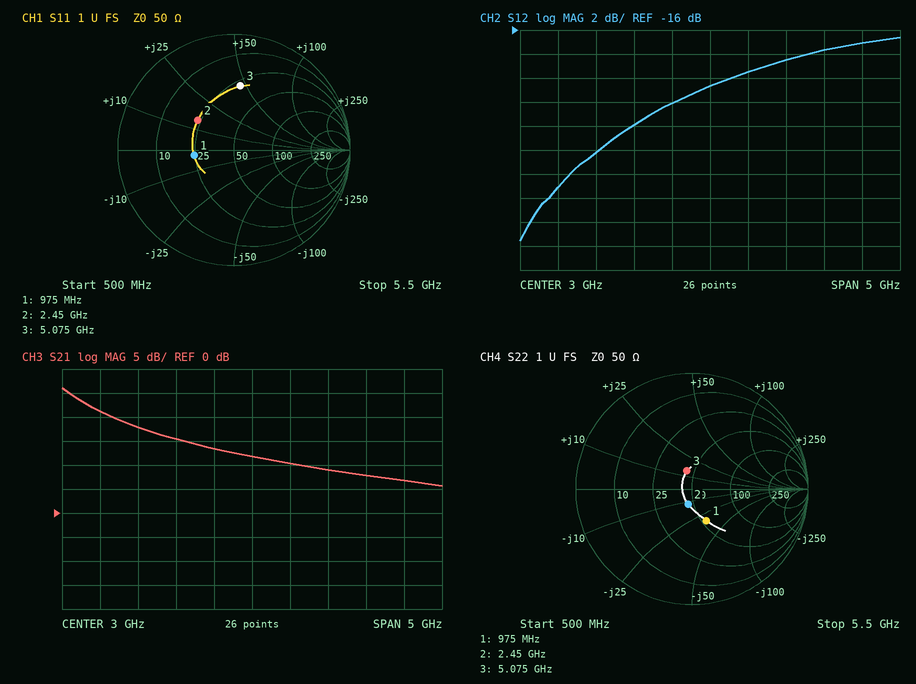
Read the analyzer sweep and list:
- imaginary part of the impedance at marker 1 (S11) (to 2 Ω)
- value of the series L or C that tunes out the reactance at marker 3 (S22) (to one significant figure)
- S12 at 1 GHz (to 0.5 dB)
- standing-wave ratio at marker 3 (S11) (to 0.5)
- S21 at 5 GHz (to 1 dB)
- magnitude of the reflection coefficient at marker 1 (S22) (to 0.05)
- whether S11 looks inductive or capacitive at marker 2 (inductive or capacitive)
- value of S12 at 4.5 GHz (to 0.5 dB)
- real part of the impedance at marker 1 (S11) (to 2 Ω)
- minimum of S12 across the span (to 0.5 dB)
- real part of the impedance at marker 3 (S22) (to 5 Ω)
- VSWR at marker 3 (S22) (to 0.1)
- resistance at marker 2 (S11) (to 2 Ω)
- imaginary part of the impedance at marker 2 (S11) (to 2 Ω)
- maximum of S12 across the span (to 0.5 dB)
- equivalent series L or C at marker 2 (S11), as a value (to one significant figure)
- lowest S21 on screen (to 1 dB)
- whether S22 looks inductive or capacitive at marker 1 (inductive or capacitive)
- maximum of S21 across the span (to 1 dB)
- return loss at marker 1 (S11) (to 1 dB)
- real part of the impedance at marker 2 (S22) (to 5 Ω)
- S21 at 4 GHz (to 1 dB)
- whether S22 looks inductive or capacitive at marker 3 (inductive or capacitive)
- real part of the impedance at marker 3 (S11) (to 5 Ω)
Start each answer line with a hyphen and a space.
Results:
- -2 Ω
- 2 pF
- -29.0 dB
- 3.5
- 7 dB
- 0.30
- inductive
- -17.5 dB
- 24 Ω
- -33.5 dB
- 45 Ω
- 1.4
- 24 Ω
- +14 Ω
- -16.5 dB
- 900 pH
- 6 dB
- capacitive
- 26 dB
- 9 dB
- 45 Ω
- 9 dB
- inductive
- 30 Ω
